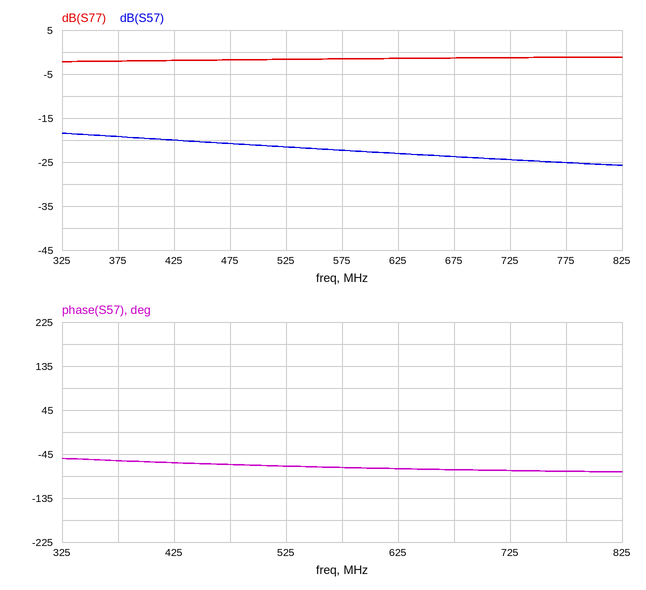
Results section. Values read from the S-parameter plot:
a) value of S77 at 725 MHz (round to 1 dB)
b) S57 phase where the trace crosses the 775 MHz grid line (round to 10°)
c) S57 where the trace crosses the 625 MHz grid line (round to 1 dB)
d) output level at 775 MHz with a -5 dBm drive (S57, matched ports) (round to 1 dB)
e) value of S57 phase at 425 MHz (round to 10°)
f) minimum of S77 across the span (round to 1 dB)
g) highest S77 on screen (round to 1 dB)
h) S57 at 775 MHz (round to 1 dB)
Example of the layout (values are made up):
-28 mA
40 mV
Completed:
-1 dB
-80°
-23 dB
-30 dBm
-60°
-2 dB
-1 dB
-25 dB
